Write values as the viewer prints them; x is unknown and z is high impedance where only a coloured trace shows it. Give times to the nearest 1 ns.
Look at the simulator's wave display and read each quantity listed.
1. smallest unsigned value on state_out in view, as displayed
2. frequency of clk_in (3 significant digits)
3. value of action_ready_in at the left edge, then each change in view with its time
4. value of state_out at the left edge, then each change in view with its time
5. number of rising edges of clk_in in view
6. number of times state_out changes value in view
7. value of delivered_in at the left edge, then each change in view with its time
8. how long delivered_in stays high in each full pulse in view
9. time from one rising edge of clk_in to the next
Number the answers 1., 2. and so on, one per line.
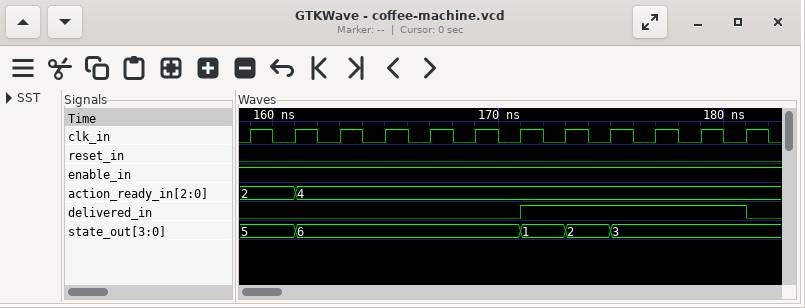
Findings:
1. 1
2. 500 MHz
3. 2, 4 at 161 ns
4. 5, 6 at 161 ns, 1 at 171 ns, 2 at 173 ns, 3 at 175 ns
5. 12
6. 4
7. 0, 1 at 171 ns, 0 at 181 ns
8. 10 ns
9. 2 ns
